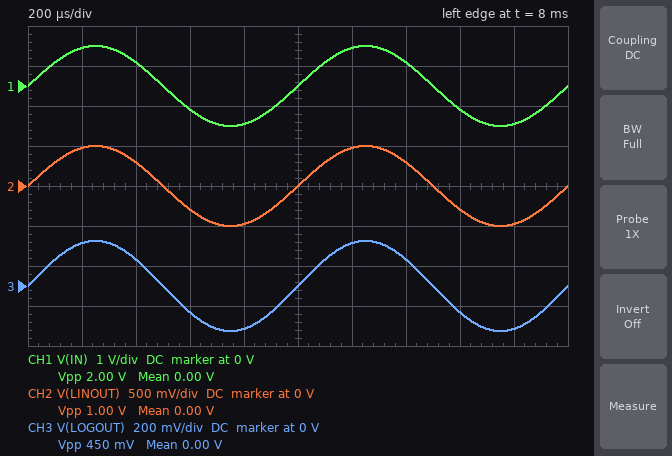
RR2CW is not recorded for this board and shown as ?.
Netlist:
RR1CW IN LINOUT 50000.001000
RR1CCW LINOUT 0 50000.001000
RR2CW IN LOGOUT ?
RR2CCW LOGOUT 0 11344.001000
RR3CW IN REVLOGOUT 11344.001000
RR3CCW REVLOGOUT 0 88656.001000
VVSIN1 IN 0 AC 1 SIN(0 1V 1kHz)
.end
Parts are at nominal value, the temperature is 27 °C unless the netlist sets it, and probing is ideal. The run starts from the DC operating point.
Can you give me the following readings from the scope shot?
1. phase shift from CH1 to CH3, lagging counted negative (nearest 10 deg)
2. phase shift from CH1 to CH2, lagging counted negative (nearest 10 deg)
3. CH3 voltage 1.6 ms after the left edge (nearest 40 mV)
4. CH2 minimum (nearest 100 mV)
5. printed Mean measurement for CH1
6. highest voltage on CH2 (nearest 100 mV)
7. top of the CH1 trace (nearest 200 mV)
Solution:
0 deg
0 deg
-120 mV
-500 mV
0.00 V
500 mV
1.0 V
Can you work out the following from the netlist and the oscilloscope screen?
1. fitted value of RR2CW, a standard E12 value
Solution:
39 kΩ
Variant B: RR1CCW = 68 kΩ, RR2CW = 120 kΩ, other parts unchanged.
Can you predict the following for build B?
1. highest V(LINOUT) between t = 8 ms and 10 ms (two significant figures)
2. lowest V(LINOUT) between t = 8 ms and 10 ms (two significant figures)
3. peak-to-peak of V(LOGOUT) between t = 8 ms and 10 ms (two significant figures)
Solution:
580 mV
-580 mV
170 mV
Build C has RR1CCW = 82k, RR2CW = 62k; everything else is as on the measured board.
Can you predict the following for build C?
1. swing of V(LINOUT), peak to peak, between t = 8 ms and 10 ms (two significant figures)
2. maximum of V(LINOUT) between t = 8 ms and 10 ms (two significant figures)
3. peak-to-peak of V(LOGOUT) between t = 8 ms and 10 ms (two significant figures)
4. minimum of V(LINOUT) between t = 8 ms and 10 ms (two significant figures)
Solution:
1.2 V
620 mV
310 mV
-620 mV
